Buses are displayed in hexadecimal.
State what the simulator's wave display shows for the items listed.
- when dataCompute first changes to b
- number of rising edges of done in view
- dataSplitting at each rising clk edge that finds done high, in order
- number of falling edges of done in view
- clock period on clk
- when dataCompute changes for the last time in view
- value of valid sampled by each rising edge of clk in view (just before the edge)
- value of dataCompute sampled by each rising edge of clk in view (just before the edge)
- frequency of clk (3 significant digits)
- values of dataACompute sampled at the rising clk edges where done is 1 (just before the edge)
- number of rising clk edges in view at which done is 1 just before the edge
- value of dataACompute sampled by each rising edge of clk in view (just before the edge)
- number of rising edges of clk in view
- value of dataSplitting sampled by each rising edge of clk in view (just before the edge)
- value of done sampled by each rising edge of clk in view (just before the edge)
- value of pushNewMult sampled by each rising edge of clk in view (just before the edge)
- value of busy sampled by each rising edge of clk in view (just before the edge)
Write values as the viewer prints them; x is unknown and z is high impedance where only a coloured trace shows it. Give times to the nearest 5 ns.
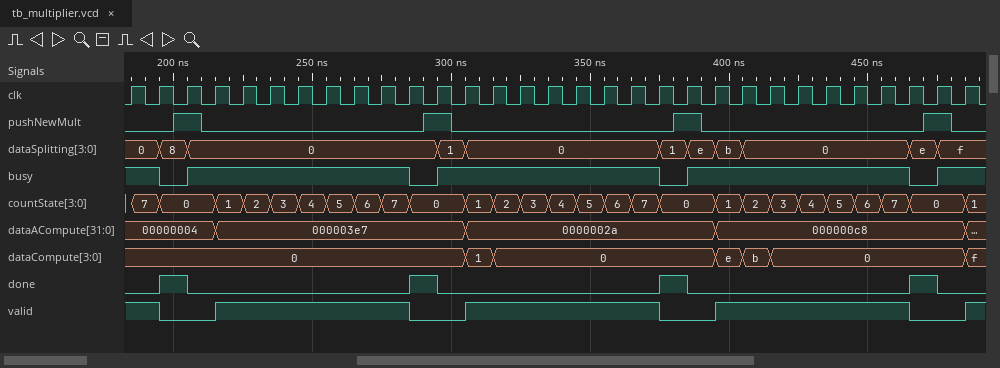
405 ns
4
8, 0, 1, e
4
10 ns
485 ns
1 1 0 0 1 1 1 1 1 1 1 0 0 1 1 1 1 1 1 1 0 0 1 1 1 1 1 1 1 0 0
0, 0, 0, 0, 0, 0, 0, 0, 0, 0, 0, 0, 0, 1, 0, 0, 0, 0, 0, 0, 0, 0, e, b, 0, 0, 0, 0, 0, 0, 0
100 MHz
00000004, 000003e7, 0000002a, 000000c8
4
00000004, 00000004, 00000004, 00000004, 000003e7, 000003e7, 000003e7, 000003e7, 000003e7, 000003e7, 000003e7, 000003e7, 000003e7, 0000002a, 0000002a, 0000002a, 0000002a, 0000002a, 0000002a, 0000002a, 0000002a, 0000002a, 000000c8, 000000c8, 000000c8, 000000c8, 000000c8, 000000c8, 000000c8, 000000c8, 000000c8
31
0, 0, 8, 0, 0, 0, 0, 0, 0, 0, 0, 0, 1, 0, 0, 0, 0, 0, 0, 0, 1, e, b, 0, 0, 0, 0, 0, 0, e, f
0 0 1 0 0 0 0 0 0 0 0 1 0 0 0 0 0 0 0 0 1 0 0 0 0 0 0 0 0 1 0
0 0 1 0 0 0 0 0 0 0 0 1 0 0 0 0 0 0 0 0 1 0 0 0 0 0 0 0 0 1 0
1 1 0 1 1 1 1 1 1 1 1 0 1 1 1 1 1 1 1 1 0 1 1 1 1 1 1 1 1 0 1
